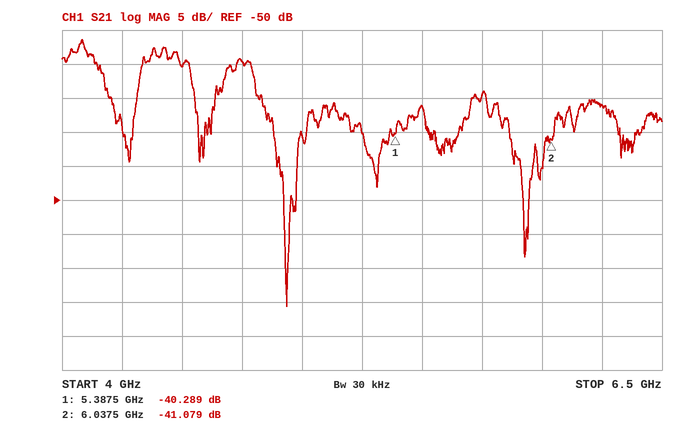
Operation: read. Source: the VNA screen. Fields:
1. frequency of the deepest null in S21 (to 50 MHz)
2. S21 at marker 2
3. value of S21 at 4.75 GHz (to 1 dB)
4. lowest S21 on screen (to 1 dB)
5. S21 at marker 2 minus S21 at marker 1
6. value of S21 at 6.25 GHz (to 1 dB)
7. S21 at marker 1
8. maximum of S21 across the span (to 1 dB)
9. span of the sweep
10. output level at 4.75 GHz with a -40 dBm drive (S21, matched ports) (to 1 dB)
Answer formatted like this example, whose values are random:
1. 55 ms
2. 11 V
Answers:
1. 4.95 GHz
2. -41.079 dB
3. -30 dB
4. -66 dB
5. -0.790 dB
6. -36 dB
7. -40.289 dB
8. -26 dB
9. 2.5 GHz
10. -70 dBm
